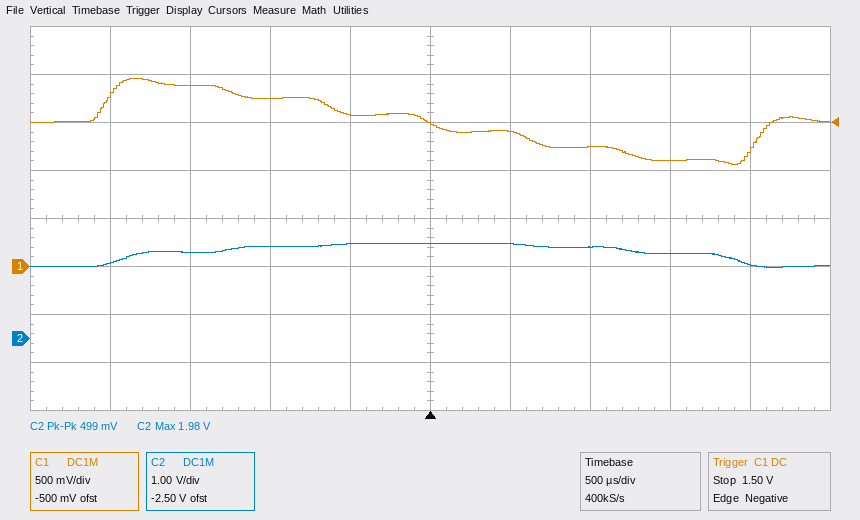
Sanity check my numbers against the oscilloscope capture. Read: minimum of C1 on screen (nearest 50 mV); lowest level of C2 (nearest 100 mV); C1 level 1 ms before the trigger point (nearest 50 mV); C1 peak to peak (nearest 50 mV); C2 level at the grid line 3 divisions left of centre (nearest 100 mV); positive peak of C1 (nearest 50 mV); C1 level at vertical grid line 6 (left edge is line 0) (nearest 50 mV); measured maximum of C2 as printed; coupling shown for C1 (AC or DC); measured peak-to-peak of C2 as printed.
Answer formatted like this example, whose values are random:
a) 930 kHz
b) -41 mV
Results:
a) 1.05 V
b) 1.5 V
c) 1.75 V
d) 900 mV
e) 1.8 V
f) 1.95 V
g) 1.40 V
h) 1.98 V
i) DC
j) 499 mV
